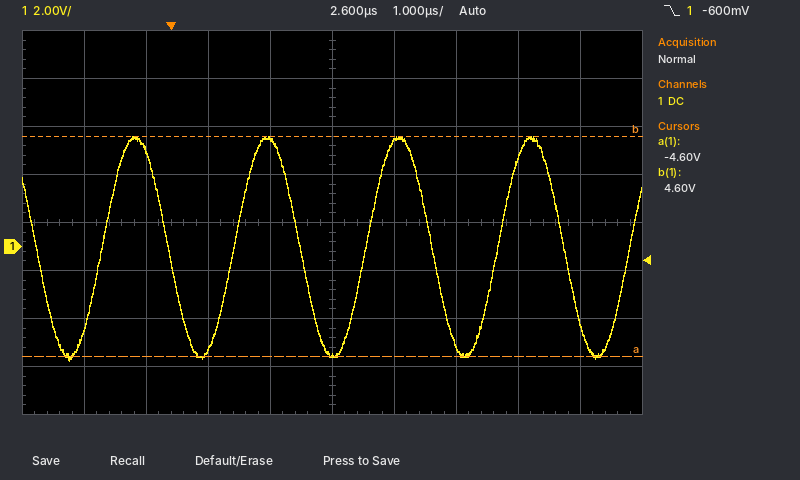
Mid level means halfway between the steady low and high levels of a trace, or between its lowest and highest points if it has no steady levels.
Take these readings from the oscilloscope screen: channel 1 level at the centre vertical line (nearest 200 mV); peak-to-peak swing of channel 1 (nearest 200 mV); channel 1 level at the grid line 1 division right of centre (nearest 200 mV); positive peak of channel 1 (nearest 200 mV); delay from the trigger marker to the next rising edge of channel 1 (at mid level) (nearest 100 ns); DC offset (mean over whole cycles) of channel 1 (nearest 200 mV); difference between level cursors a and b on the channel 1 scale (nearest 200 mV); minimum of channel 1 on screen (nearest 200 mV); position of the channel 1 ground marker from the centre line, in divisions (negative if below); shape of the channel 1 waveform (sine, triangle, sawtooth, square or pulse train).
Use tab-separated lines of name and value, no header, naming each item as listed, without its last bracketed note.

channel 1 level at the centre vertical line	-4.6 V
peak-to-peak swing of channel 1	9.4 V
channel 1 level at the grid line 1 division right of centre	4.4 V
positive peak of channel 1	4.6 V
delay from the trigger marker to the next rising edge of channel 1 (at mid level)	1.0 µs
DC offset (mean over whole cycles) of channel 1	0.0 V
difference between level cursors a and b on the channel 1 scale	9.2 V
minimum of channel 1 on screen	-4.8 V
position of the channel 1 ground marker from the centre line, in divisions	-0.5 div
shape of the channel 1 waveform	sine
